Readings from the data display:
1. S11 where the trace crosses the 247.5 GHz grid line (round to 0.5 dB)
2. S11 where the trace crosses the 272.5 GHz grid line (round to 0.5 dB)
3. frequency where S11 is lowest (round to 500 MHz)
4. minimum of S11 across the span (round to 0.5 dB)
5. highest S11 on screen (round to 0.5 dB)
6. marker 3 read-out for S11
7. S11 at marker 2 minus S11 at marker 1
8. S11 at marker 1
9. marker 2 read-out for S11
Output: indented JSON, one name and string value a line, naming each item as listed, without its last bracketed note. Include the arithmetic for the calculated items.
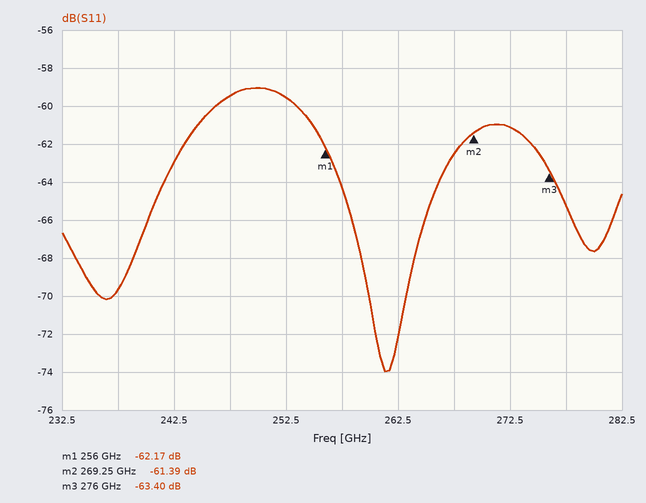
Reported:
{
  "S11 where the trace crosses the 247.5 GHz grid line": "-59.5 dB",
  "S11 where the trace crosses the 272.5 GHz grid line": "-61.0 dB",
  "frequency where S11 is lowest": "261.5 GHz",
  "minimum of S11 across the span": "-74.0 dB",
  "highest S11 on screen": "-59.0 dB",
  "marker 3 read-out for S11": "-63.40 dB",
  "S11 at marker 2 minus S11 at marker 1": "-61.39 − (-62.17) = 0.78 dB",
  "S11 at marker 1": "-62.17 dB",
  "marker 2 read-out for S11": "-61.39 dB"
}
